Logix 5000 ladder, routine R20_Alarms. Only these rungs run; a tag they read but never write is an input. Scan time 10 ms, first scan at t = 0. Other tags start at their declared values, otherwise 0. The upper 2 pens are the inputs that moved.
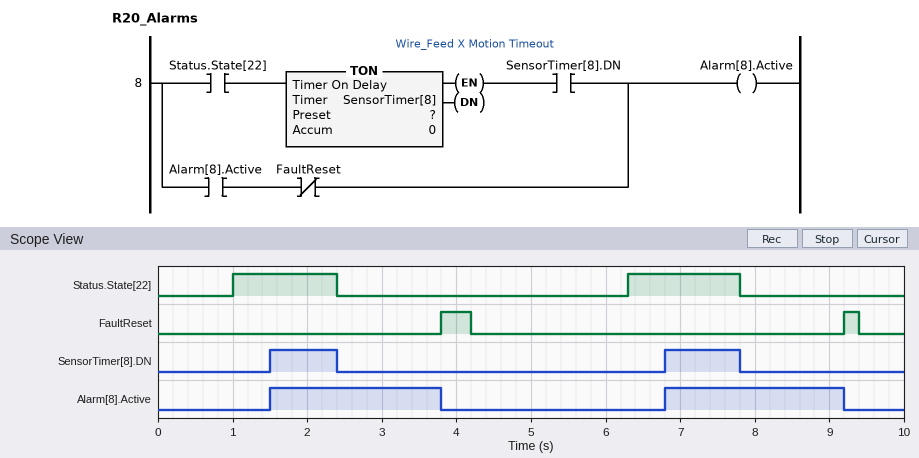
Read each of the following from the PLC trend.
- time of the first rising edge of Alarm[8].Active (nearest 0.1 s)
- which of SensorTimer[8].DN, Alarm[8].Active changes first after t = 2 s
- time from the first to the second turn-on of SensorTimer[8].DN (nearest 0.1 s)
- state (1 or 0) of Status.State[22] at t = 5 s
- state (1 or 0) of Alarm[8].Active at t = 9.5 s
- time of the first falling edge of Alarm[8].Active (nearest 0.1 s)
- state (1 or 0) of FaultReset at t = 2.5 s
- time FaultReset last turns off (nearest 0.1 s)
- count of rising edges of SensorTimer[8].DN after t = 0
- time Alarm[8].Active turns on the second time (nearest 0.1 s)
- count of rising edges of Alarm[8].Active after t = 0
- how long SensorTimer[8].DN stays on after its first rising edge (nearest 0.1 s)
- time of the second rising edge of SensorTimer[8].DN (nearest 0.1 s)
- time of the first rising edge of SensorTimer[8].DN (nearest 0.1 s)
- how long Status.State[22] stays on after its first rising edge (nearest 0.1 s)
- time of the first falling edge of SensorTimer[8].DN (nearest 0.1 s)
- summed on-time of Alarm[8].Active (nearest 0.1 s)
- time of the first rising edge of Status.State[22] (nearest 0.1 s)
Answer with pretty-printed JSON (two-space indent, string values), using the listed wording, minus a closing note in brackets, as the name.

{
  "time of the first rising edge of Alarm[8].Active": "1.5 s",
  "which of SensorTimer[8].DN, Alarm[8].Active changes first after t = 2 s": "SensorTimer[8].DN",
  "time from the first to the second turn-on of SensorTimer[8].DN": "5.3 s",
  "state (1 or 0) of Status.State[22] at t = 5 s": "0",
  "state (1 or 0) of Alarm[8].Active at t = 9.5 s": "0",
  "time of the first falling edge of Alarm[8].Active": "3.8 s",
  "state (1 or 0) of FaultReset at t = 2.5 s": "0",
  "time FaultReset last turns off": "9.4 s",
  "count of rising edges of SensorTimer[8].DN after t = 0": "2",
  "time Alarm[8].Active turns on the second time": "6.8 s",
  "count of rising edges of Alarm[8].Active after t = 0": "2",
  "how long SensorTimer[8].DN stays on after its first rising edge": "0.9 s",
  "time of the second rising edge of SensorTimer[8].DN": "6.8 s",
  "time of the first rising edge of SensorTimer[8].DN": "1.5 s",
  "how long Status.State[22] stays on after its first rising edge": "1.4 s",
  "time of the first falling edge of SensorTimer[8].DN": "2.4 s",
  "summed on-time of Alarm[8].Active": "4.7 s",
  "time of the first rising edge of Status.State[22]": "1.0 s"
}
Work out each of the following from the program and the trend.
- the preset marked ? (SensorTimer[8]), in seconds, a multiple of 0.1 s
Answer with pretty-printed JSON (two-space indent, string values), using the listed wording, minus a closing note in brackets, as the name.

{
  "the preset marked ? (SensorTimer[8]), in seconds, a multiple of 0.1 s": "0.5 s"
}
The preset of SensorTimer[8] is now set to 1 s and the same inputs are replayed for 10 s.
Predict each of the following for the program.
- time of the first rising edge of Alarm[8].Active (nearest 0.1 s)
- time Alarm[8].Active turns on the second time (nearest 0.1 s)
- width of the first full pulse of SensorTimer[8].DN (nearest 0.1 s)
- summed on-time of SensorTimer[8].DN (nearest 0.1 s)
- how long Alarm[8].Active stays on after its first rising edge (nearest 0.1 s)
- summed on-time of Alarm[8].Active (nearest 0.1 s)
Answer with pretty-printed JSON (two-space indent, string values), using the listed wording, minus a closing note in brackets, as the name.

{
  "time of the first rising edge of Alarm[8].Active": "2.0 s",
  "time Alarm[8].Active turns on the second time": "7.3 s",
  "width of the first full pulse of SensorTimer[8].DN": "0.4 s",
  "summed on-time of SensorTimer[8].DN": "0.9 s",
  "how long Alarm[8].Active stays on after its first rising edge": "1.8 s",
  "summed on-time of Alarm[8].Active": "3.7 s"
}
